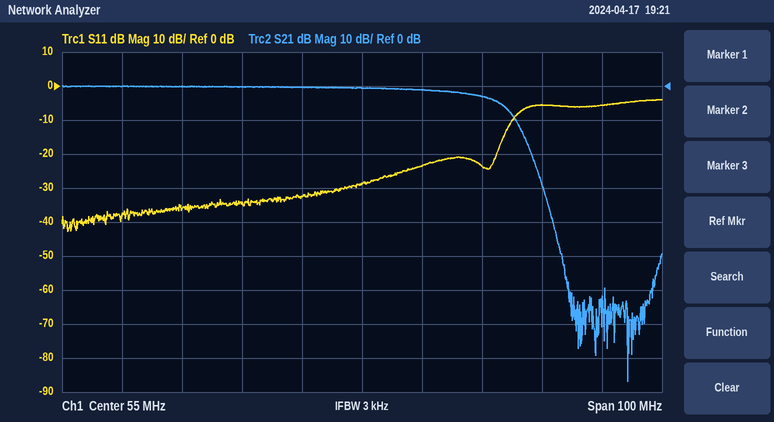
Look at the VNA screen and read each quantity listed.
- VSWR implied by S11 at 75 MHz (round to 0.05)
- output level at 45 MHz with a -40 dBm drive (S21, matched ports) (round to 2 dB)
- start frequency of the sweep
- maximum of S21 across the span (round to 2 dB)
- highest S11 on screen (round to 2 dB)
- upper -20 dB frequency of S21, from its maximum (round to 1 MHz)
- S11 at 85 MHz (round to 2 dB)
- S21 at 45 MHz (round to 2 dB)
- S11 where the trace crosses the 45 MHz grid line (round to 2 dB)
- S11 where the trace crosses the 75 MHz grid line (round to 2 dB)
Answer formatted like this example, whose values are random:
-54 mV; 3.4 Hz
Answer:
1.15; -40 dBm; 5 MHz; 0 dB; -4 dB; 83 MHz; -6 dB; 0 dB; -32 dB; -24 dB
